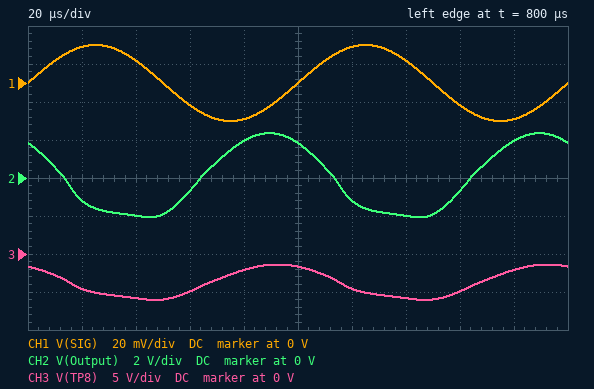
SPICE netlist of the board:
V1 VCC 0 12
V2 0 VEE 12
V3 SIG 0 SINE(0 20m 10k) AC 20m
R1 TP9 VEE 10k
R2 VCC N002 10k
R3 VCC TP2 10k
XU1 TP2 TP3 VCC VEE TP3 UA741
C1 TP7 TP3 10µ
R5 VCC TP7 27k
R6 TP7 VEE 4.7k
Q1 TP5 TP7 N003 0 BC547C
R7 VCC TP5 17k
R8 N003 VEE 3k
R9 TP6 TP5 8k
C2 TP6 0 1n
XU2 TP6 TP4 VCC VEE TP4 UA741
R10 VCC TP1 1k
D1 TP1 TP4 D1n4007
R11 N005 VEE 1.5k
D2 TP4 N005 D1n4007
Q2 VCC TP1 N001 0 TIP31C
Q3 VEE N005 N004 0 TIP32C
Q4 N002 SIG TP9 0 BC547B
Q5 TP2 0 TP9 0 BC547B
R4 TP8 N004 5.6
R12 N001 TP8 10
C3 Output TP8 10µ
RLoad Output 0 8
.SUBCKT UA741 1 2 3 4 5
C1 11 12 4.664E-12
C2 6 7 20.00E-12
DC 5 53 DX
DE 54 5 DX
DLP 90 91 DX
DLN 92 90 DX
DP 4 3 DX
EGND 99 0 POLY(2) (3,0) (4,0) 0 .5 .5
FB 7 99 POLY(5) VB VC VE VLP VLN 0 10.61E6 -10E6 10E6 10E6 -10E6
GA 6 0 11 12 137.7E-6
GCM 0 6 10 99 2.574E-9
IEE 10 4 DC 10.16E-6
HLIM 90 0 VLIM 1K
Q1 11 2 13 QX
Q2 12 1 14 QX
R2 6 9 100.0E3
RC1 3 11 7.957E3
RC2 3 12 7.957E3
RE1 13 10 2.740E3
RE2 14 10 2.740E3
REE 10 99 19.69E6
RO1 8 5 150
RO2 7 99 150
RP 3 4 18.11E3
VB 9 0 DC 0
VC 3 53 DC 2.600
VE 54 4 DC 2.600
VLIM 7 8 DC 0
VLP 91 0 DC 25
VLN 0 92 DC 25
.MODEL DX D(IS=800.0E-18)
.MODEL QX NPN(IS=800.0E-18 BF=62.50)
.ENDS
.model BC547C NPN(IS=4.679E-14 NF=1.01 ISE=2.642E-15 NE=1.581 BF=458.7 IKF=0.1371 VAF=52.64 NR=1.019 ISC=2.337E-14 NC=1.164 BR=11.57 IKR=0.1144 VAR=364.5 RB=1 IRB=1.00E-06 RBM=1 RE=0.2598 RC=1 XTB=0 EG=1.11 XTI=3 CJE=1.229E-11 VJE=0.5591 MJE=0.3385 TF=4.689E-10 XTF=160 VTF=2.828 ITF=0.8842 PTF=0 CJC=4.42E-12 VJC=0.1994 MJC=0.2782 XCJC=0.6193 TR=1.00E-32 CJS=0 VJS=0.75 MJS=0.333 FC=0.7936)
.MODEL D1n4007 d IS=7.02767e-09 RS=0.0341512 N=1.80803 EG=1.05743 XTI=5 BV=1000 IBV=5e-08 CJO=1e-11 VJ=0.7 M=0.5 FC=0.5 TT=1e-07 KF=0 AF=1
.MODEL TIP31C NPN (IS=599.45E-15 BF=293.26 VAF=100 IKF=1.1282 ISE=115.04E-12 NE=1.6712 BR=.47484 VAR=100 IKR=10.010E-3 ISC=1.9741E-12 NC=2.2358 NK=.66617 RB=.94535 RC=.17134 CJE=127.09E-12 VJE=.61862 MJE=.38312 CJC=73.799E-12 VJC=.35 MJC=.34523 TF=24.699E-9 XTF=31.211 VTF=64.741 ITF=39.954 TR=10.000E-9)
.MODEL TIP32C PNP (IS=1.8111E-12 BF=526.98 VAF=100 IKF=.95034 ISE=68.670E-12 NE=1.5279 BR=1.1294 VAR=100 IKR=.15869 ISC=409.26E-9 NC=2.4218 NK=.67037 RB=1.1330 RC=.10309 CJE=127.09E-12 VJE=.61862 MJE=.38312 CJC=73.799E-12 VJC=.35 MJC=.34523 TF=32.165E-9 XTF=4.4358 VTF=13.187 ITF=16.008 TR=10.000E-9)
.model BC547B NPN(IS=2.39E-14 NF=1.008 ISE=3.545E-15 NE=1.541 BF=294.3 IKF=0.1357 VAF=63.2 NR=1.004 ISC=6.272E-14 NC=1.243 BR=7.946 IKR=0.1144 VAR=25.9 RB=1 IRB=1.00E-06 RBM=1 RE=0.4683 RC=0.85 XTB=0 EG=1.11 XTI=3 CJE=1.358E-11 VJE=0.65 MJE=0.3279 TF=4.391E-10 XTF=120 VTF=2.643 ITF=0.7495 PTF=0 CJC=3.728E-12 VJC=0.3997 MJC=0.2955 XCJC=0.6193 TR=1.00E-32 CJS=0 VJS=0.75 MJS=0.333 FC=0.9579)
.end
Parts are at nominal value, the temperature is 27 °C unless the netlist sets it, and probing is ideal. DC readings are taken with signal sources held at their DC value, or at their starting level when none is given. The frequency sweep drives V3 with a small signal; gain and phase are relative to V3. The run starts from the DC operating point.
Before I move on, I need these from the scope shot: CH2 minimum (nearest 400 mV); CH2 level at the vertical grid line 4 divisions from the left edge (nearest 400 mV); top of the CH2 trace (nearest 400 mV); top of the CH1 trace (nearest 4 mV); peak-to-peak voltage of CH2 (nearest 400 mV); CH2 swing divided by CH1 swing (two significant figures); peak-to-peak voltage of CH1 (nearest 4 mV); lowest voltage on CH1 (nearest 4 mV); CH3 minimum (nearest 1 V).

-2.0 V
2.0 V
2.4 V
20 mV
4.4 V
110
40 mV
-20 mV
-6 V
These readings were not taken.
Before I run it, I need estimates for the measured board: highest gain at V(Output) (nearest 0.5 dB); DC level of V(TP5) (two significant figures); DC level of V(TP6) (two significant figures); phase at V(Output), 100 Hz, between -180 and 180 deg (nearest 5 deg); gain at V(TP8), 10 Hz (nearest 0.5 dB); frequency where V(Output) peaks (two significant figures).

49.0 dB
-4.6 V
-4.6 V
-95 deg
54.0 dB
2.8 kHz
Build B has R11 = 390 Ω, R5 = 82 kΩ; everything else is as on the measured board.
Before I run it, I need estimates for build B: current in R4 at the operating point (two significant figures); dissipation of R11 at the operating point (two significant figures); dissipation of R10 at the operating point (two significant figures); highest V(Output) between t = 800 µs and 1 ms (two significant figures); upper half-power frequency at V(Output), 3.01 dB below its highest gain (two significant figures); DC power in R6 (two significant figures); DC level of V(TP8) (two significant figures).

12 mA
470 mW
83 mW
39 mV
8.1 kHz
360 µW
2.2 V
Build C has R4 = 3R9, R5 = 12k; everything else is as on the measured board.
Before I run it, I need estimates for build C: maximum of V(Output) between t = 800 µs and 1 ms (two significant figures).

400 mV
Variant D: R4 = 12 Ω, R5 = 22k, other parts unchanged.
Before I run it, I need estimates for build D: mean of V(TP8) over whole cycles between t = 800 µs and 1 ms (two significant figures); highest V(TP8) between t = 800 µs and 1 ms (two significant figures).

-4.9 V
-3.3 V
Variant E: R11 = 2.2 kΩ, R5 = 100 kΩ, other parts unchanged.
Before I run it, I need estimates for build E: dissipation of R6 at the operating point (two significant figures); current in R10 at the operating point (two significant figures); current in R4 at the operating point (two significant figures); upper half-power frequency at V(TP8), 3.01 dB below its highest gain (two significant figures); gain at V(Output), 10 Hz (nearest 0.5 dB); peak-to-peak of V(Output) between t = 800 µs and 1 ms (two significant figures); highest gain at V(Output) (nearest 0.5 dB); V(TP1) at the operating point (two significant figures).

250 µW
2.3 mA
6.0 mA
1.7 kHz
8.0 dB
3.6 V
48.0 dB
9.7 V
